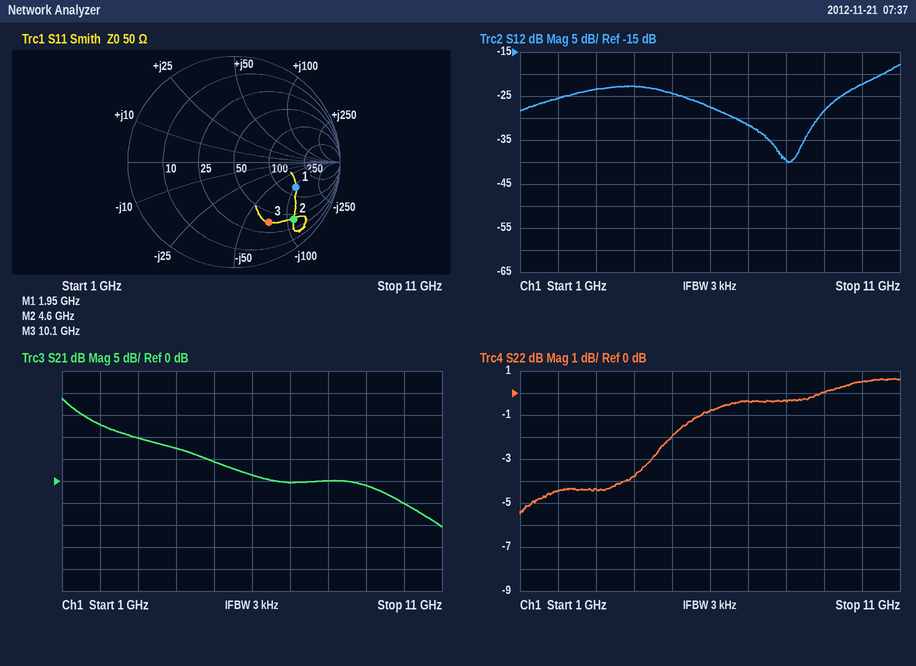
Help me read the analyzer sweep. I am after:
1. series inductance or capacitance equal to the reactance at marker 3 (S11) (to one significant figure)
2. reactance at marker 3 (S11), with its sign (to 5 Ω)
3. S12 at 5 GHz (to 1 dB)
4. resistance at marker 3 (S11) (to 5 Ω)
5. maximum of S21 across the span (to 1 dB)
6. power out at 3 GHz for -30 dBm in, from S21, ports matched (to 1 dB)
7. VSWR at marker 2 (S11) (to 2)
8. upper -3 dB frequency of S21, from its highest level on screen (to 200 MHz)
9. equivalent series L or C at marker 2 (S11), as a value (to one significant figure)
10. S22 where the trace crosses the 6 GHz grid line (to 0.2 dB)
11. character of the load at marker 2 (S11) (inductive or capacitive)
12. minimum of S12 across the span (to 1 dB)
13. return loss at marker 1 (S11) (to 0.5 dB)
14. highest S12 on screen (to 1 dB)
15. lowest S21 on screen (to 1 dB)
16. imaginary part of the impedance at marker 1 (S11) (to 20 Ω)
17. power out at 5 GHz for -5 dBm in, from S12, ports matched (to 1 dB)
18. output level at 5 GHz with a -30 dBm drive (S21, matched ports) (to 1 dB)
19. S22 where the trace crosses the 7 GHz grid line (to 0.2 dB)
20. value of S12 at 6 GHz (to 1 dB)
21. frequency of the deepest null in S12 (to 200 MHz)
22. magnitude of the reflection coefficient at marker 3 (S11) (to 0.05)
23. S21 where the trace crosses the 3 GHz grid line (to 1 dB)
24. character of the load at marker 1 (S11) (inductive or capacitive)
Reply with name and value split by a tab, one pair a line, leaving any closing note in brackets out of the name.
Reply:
series inductance or capacitance equal to the reactance at marker 3 (S11)	200 fF
reactance at marker 3 (S11), with its sign	-75 Ω
S12 at 5 GHz	-24 dB
resistance at marker 3 (S11)	35 Ω
maximum of S21 across the span	19 dB
power out at 3 GHz for -30 dBm in, from S21, ports matched	-20 dBm
VSWR at marker 2 (S11)	8
upper -3 dB frequency of S21, from its highest level on screen	1.4 GHz
equivalent series L or C at marker 2 (S11), as a value	300 fF
S22 where the trace crosses the 6 GHz grid line	-0.8 dB
character of the load at marker 2 (S11)	capacitive
minimum of S12 across the span	-40 dB
return loss at marker 1 (S11)	4.0 dB
highest S12 on screen	-18 dB
lowest S21 on screen	-10 dB
imaginary part of the impedance at marker 1 (S11)	-100 Ω
power out at 5 GHz for -5 dBm in, from S12, ports matched	-29 dBm
output level at 5 GHz with a -30 dBm drive (S21, matched ports)	-26 dBm
S22 where the trace crosses the 7 GHz grid line	-0.4 dB
value of S12 at 6 GHz	-27 dB
frequency of the deepest null in S12	8.0 GHz
magnitude of the reflection coefficient at marker 3 (S11)	0.65
S21 where the trace crosses the 3 GHz grid line	10 dB
character of the load at marker 1 (S11)	capacitive
